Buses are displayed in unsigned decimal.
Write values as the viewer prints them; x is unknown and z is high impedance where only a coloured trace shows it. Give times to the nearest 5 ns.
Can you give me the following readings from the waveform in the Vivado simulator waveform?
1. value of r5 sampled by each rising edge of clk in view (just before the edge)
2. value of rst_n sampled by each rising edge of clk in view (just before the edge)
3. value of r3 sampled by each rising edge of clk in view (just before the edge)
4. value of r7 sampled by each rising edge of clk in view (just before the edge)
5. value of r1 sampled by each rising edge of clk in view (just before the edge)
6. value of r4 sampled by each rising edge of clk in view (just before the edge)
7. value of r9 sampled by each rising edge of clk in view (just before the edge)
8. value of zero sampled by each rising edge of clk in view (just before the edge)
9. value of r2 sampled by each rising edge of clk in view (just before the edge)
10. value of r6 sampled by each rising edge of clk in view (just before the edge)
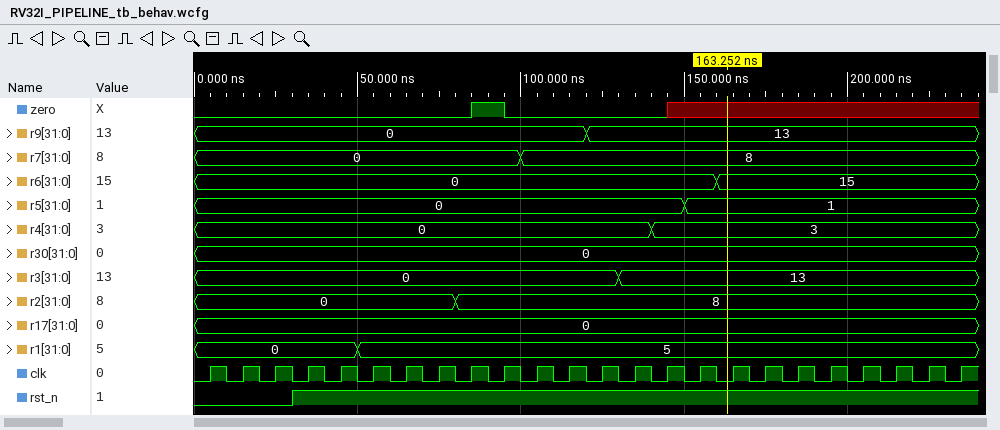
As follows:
0, 0, 0, 0, 0, 0, 0, 0, 0, 0, 0, 0, 0, 0, 0, 1, 1, 1, 1, 1, 1, 1, 1, 1
0 0 0 1 1 1 1 1 1 1 1 1 1 1 1 1 1 1 1 1 1 1 1 1
0, 0, 0, 0, 0, 0, 0, 0, 0, 0, 0, 0, 0, 13, 13, 13, 13, 13, 13, 13, 13, 13, 13, 13
0, 0, 0, 0, 0, 0, 0, 0, 0, 0, 8, 8, 8, 8, 8, 8, 8, 8, 8, 8, 8, 8, 8, 8
0, 0, 0, 0, 0, 5, 5, 5, 5, 5, 5, 5, 5, 5, 5, 5, 5, 5, 5, 5, 5, 5, 5, 5
0, 0, 0, 0, 0, 0, 0, 0, 0, 0, 0, 0, 0, 0, 3, 3, 3, 3, 3, 3, 3, 3, 3, 3
0, 0, 0, 0, 0, 0, 0, 0, 0, 0, 0, 0, 13, 13, 13, 13, 13, 13, 13, 13, 13, 13, 13, 13
0 0 0 0 0 0 0 0 0 1 0 0 0 0 0 x x x x x x x x x
0, 0, 0, 0, 0, 0, 0, 0, 8, 8, 8, 8, 8, 8, 8, 8, 8, 8, 8, 8, 8, 8, 8, 8
0, 0, 0, 0, 0, 0, 0, 0, 0, 0, 0, 0, 0, 0, 0, 0, 15, 15, 15, 15, 15, 15, 15, 15
